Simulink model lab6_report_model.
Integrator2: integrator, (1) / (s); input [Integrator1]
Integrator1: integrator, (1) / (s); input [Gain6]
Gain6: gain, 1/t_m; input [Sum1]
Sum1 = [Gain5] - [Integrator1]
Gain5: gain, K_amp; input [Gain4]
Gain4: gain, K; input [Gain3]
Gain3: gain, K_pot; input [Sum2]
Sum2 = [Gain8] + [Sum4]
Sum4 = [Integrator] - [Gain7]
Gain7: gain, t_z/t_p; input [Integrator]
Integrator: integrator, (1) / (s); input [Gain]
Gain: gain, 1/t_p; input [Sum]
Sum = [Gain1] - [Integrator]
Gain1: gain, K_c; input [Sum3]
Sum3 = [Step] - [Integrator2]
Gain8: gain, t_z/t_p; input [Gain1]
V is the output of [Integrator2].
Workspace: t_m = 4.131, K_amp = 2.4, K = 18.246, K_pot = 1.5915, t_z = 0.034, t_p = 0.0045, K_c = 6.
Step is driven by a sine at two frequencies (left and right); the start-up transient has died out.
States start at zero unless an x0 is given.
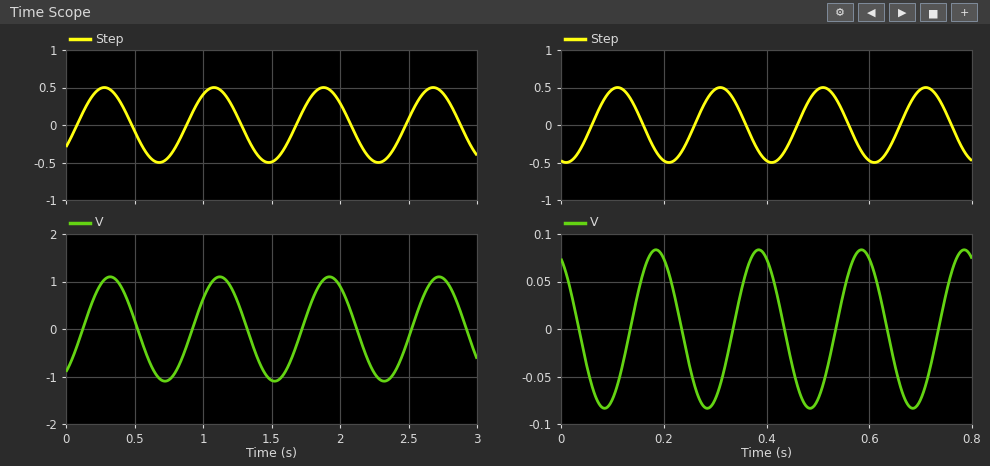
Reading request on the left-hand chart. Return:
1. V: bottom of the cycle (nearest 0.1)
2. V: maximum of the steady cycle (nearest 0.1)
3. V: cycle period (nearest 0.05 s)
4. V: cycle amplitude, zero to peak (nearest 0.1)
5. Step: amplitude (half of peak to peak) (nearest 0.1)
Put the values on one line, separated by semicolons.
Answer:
-1.1; 1.1; 0.80 s; 1.1; 0.5
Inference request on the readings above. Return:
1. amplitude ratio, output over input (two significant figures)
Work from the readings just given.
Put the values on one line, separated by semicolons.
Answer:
2.2
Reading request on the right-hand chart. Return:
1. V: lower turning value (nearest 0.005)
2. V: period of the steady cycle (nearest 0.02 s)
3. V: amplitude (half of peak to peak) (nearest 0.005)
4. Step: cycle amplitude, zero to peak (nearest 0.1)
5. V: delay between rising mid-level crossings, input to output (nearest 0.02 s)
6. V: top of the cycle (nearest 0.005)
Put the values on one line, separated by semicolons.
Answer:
-0.085; 0.20 s; 0.085; 0.5; 0.08 s; 0.085
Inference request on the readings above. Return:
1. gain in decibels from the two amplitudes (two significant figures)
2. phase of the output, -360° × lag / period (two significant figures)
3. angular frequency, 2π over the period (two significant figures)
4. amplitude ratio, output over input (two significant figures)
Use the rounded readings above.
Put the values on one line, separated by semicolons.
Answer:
-15 dB; -140°; 31 rad/s; 0.17
